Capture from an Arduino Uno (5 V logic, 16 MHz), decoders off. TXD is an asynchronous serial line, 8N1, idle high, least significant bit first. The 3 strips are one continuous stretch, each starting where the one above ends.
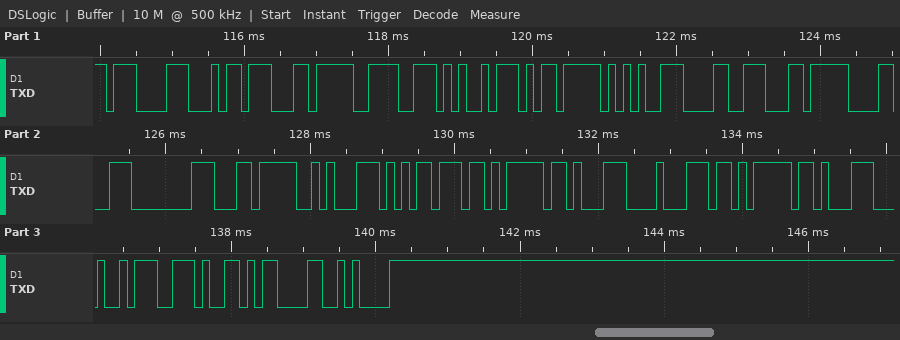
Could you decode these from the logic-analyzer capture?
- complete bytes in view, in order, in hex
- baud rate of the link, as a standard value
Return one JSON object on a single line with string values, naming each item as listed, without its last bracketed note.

{"complete bytes in view, in order, in hex": "87 B4 EC 9E A5 ED 95 98 EC 98 80 EC 8A B5 EB 8B 88 EB 8B A4 2E 0D 0A", "baud rate of the link, as a standard value": "9600 baud"}
